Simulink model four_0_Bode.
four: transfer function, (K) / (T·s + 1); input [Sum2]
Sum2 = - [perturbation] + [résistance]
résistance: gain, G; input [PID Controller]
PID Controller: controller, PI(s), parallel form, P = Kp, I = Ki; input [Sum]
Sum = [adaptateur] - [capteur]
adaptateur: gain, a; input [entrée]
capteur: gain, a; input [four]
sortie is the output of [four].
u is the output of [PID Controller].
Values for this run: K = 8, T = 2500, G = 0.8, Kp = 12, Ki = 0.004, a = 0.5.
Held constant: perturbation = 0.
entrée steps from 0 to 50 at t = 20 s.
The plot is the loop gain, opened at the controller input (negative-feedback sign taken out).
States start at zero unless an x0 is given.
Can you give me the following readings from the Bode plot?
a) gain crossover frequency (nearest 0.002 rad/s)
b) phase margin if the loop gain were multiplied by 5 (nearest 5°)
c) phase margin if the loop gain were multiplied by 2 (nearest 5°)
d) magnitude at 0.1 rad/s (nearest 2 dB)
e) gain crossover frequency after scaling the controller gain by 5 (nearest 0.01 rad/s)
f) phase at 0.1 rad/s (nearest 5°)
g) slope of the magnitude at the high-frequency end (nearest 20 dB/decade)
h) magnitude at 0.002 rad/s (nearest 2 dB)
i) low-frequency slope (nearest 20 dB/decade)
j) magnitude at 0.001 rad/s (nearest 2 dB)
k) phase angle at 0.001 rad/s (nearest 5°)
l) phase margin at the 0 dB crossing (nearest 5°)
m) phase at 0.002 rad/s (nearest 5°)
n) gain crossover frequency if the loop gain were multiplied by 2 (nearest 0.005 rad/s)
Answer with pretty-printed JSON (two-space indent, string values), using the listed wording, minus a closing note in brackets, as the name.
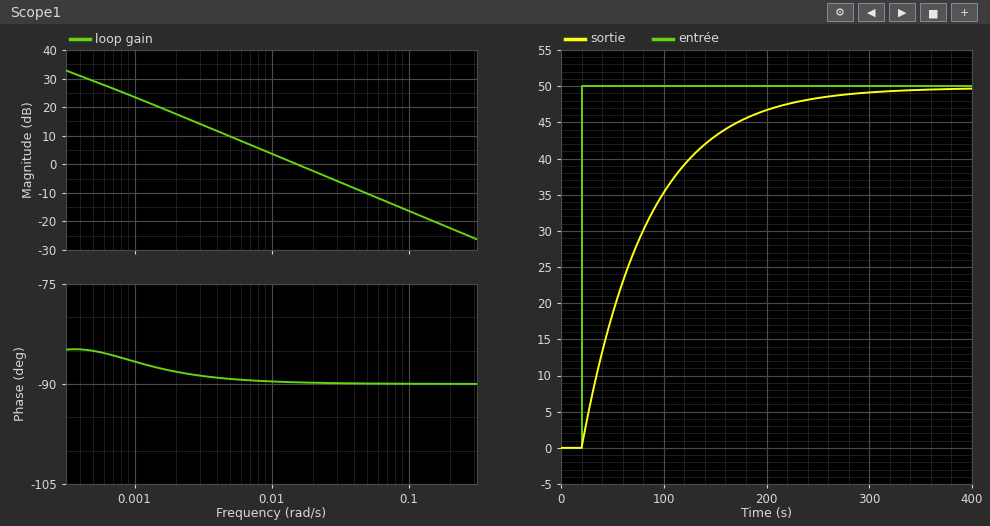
{
  "gain crossover frequency": "0.016 rad/s",
  "phase margin if the loop gain were multiplied by 5": "90°",
  "phase margin if the loop gain were multiplied by 2": "90°",
  "magnitude at 0.1 rad/s": "-16 dB",
  "gain crossover frequency after scaling the controller gain by 5": "0.08 rad/s",
  "phase at 0.1 rad/s": "-90°",
  "slope of the magnitude at the high-frequency end": "-20 dB/decade",
  "magnitude at 0.002 rad/s": "18 dB",
  "low-frequency slope": "-20 dB/decade",
  "magnitude at 0.001 rad/s": "24 dB",
  "phase angle at 0.001 rad/s": "-85°",
  "phase margin at the 0 dB crossing": "90°",
  "phase at 0.002 rad/s": "-90°",
  "gain crossover frequency if the loop gain were multiplied by 2": "0.030 rad/s"
}
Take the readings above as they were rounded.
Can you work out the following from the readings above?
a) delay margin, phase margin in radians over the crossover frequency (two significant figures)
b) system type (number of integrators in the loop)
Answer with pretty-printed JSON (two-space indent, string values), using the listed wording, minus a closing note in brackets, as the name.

{
  "delay margin, phase margin in radians over the crossover frequency": "98 s",
  "system type": "1"
}
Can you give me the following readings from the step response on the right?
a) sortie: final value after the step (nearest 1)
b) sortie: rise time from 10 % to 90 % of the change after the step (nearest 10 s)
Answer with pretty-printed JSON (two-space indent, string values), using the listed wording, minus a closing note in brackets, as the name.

{
  "sortie: final value after the step": "50",
  "sortie: rise time from 10 % to 90 % of the change after the step": "140 s"
}
